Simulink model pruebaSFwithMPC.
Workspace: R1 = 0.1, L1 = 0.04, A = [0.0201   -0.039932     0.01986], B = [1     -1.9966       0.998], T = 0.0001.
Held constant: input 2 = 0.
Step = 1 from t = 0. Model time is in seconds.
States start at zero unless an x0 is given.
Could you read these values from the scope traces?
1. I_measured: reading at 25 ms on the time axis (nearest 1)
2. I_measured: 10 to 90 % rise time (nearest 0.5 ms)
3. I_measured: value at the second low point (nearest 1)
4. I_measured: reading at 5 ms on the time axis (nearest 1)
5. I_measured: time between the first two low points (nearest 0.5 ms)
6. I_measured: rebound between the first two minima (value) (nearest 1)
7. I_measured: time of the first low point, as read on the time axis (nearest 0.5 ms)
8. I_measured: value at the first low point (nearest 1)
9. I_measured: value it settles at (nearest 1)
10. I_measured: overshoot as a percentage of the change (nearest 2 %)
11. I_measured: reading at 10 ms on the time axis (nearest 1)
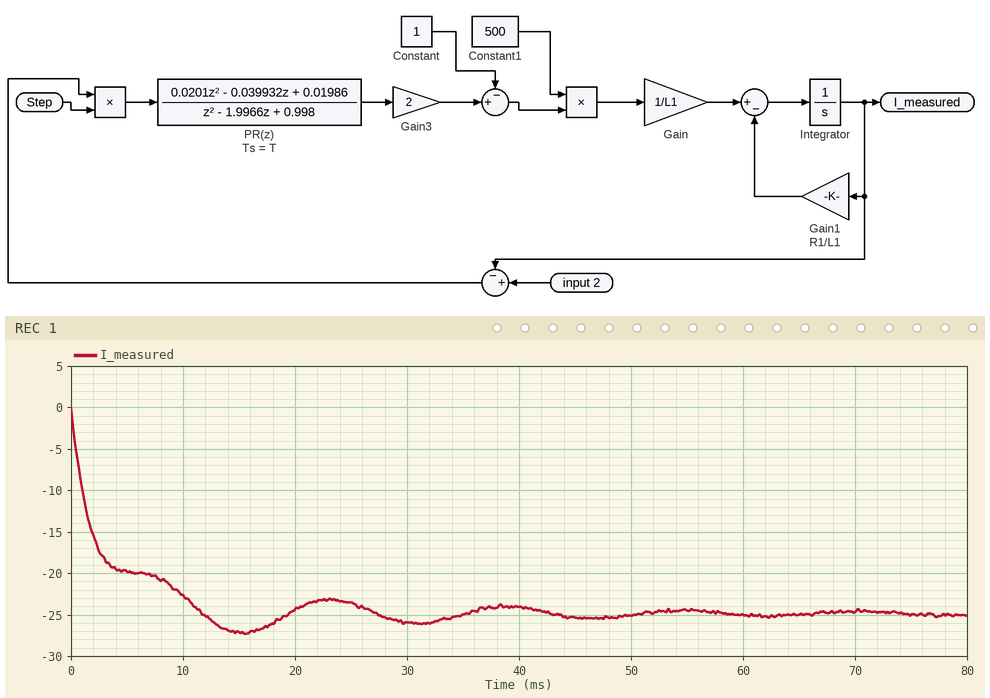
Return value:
-24
9.5 ms
-26
-20
15.5 ms
-23
15.5 ms
-27
-25
10 %
-23
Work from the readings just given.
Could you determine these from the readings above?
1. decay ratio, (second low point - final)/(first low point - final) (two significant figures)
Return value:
0.50
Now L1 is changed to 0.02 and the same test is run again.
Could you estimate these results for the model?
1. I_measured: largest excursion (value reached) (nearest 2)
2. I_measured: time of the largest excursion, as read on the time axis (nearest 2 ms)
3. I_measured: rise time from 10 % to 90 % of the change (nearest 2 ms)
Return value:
-28
14 ms
8 ms
